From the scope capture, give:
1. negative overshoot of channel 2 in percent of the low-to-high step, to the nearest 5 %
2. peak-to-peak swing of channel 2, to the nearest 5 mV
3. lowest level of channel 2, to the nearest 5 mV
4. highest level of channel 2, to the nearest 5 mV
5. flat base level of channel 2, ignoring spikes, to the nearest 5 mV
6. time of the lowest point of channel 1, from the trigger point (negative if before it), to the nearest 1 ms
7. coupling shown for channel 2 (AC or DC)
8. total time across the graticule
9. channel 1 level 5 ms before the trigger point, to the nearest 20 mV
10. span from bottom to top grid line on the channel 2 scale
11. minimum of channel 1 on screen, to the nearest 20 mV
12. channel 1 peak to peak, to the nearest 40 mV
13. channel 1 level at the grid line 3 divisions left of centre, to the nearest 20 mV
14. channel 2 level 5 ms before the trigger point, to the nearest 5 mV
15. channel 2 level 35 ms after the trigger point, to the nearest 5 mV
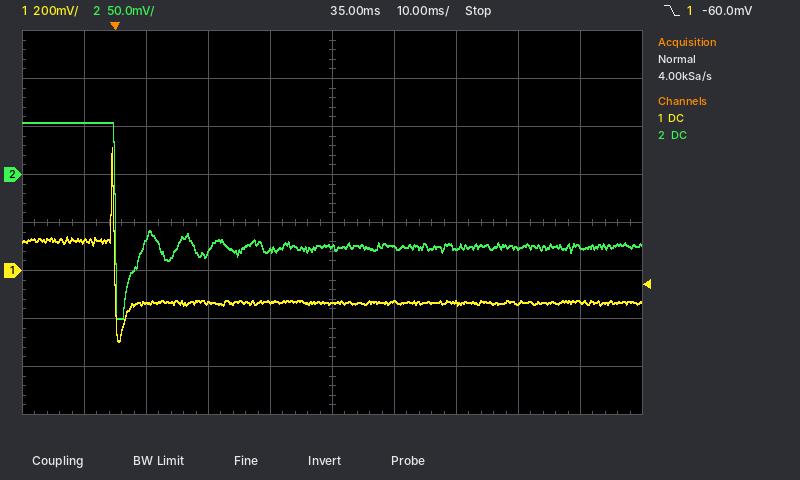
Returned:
60 %
205 mV
-150 mV
55 mV
-75 mV
+1 ms
DC
100 ms
120 mV
400 mV
-300 mV
800 mV
-140 mV
55 mV
-75 mV
